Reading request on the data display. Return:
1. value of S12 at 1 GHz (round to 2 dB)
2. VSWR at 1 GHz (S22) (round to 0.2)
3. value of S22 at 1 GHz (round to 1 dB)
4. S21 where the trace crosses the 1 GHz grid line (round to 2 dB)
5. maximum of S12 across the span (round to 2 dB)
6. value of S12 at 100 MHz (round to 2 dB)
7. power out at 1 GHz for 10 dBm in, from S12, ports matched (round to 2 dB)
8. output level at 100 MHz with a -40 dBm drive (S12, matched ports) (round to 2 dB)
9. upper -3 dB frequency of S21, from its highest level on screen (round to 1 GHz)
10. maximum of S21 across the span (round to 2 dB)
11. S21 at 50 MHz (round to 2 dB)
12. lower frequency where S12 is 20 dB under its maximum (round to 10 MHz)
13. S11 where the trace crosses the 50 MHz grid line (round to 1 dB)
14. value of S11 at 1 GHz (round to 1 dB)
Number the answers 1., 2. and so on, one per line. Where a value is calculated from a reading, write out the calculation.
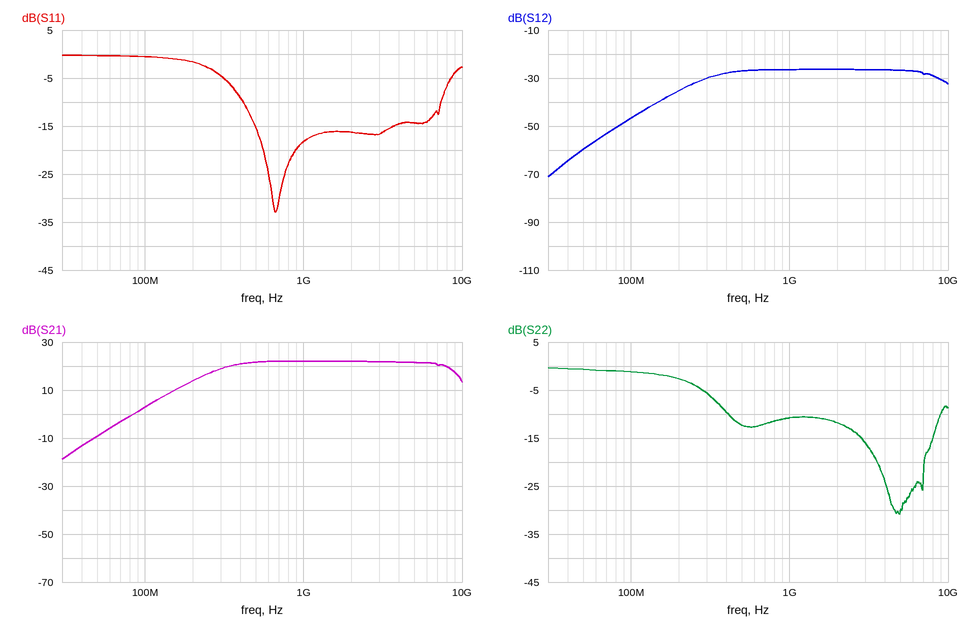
1. -26 dB
2. |Γ| = 10^(-11/20) = 0.2818; VSWR = (1 + 0.2818)/(1 − 0.2818) ≈ 1.8
3. -11 dB
4. 22 dB
5. -26 dB
6. -46 dB
7. 10 dBm + (-26 dB) = -16 dBm
8. -40 dBm + (-46 dB) = -86 dBm
9. 8 GHz
10. 22 dB
11. -10 dB
12. 100 MHz
13. 0 dB
14. -18 dB
